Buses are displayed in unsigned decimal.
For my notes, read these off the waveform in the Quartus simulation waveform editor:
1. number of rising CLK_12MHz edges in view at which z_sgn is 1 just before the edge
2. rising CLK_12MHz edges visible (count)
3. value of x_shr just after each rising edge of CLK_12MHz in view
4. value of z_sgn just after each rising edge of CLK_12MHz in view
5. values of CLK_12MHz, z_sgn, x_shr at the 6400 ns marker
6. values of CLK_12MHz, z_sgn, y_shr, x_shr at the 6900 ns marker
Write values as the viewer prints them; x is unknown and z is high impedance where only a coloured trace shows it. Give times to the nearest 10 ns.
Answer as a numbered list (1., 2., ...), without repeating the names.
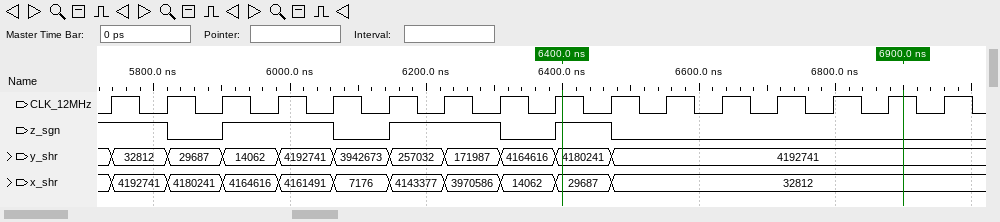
1. 7
2. 16
3. 4192741, 4180241, 4164616, 4161491, 7176, 4143377, 3970586, 14062, 29687, 32812, 32812, 32812, 32812, 32812, 32812, 32812
4. 1 0 1 1 0 1 1 0 1 0 0 0 0 0 0 0
5. CLK_12MHz=1, z_sgn=1, x_shr=29687
6. CLK_12MHz=1, z_sgn=0, y_shr=4192741, x_shr=32812
